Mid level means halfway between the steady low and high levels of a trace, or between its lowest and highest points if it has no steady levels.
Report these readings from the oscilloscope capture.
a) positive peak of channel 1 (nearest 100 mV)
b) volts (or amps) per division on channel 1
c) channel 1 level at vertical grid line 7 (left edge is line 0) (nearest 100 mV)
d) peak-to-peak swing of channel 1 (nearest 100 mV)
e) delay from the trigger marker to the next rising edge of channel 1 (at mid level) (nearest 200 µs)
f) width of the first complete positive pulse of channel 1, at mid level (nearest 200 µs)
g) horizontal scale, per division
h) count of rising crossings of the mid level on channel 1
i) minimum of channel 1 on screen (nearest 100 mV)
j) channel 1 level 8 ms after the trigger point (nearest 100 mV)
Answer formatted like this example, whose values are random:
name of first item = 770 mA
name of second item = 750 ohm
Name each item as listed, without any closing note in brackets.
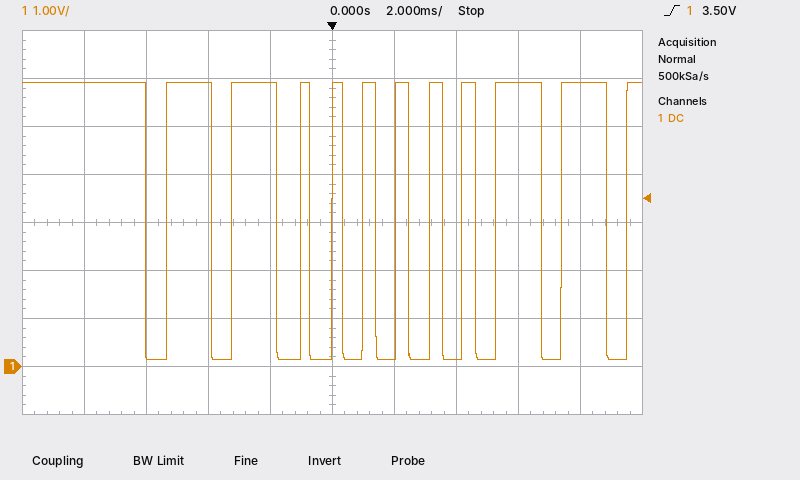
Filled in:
positive peak of channel 1 = 5.9 V
volts (or amps) per division on channel 1 = 1 V
channel 1 level at vertical grid line 7 (left edge is line 0) = 100 mV
peak-to-peak swing of channel 1 = 5.8 V
delay from the trigger marker to the next rising edge of channel 1 (at mid level) = 1.0 ms
width of the first complete positive pulse of channel 1, at mid level = 1.4 ms
horizontal scale, per division = 2 ms
count of rising crossings of the mid level on channel 1 = 11
minimum of channel 1 on screen = 100 mV
channel 1 level 8 ms after the trigger point = 5.9 V
